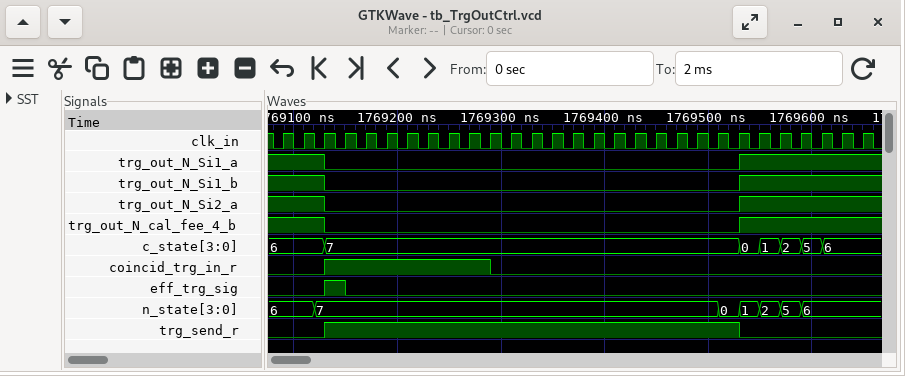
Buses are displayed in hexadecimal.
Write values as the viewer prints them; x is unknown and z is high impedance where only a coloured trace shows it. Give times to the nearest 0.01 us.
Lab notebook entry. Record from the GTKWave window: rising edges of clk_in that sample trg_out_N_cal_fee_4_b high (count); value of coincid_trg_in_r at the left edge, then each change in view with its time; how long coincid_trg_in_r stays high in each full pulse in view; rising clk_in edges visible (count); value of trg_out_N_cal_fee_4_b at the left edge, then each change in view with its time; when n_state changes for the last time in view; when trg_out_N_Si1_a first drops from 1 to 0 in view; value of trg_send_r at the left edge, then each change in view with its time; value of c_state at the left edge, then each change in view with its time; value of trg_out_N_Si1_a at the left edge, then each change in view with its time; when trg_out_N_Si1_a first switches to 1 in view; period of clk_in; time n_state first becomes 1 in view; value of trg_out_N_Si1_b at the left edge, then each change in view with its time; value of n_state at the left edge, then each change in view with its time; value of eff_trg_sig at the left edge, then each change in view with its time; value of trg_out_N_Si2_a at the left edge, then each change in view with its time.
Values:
9
0, 1 at 1769.13 us, 0 at 1769.29 us
0.16 us
29
1, 0 at 1769.13 us, 1 at 1769.53 us
1769.59 us
1769.13 us
0, 1 at 1769.13 us, 0 at 1769.53 us
6, 7 at 1769.13 us, 0 at 1769.53 us, 1 at 1769.55 us, 2 at 1769.57 us, 5 at 1769.59 us, 6 at 1769.61 us
1, 0 at 1769.13 us, 1 at 1769.53 us
1769.53 us
0.02 us
1769.53 us
1, 0 at 1769.13 us, 1 at 1769.53 us
6, 7 at 1769.12 us, 0 at 1769.51 us, 1 at 1769.53 us, 2 at 1769.55 us, 5 at 1769.57 us, 6 at 1769.59 us
0, 1 at 1769.13 us, 0 at 1769.15 us
1, 0 at 1769.13 us, 1 at 1769.53 us
